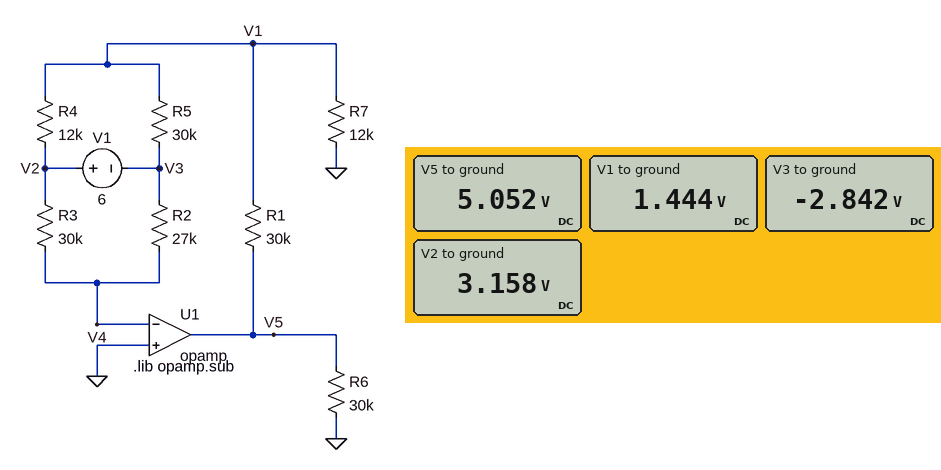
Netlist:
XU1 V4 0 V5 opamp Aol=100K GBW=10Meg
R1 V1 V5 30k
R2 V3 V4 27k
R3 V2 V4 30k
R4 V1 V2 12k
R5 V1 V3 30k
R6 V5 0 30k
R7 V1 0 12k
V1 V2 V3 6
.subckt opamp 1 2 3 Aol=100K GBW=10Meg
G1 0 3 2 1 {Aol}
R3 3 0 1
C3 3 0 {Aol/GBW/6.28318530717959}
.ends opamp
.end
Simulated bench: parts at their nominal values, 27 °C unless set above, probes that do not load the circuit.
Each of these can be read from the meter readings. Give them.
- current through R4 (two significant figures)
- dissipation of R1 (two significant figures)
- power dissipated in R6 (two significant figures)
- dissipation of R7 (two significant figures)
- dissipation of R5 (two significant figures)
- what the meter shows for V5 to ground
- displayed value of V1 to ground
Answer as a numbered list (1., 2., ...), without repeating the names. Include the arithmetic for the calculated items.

1. (3.158 V - 1.444 V) / 12 kΩ = 140 µA
2. (5.052 V - 1.444 V)^2 / 30 kΩ = 430 µW
3. (5.052 V)^2 / 30 kΩ = 850 µW
4. (1.444 V)^2 / 12 kΩ = 170 µW
5. (1.444 V - (-2.842 V))^2 / 30 kΩ = 610 µW
6. 5.052 V
7. 1.444 V
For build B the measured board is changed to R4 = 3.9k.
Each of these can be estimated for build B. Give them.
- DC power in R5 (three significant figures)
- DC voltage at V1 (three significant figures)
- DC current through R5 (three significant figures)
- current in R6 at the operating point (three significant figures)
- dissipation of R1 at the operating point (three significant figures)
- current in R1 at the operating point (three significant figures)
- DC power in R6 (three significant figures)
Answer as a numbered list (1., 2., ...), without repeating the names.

1. 940 µW
2. 2.47 V
3. 177 µA
4. 288 µA
5. 1.27 mW
6. 206 µA
7. 2.49 mW
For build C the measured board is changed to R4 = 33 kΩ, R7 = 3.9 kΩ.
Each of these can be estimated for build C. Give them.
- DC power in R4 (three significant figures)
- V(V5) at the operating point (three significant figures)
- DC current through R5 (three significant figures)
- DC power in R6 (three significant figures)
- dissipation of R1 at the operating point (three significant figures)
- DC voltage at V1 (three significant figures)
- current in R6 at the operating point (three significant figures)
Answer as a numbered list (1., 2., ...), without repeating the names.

1. 299 µW
2. 131 mV
3. 95.2 µA
4. 569 nW
5. 446 nW
6. 15.0 mV
7. 4.36 µA
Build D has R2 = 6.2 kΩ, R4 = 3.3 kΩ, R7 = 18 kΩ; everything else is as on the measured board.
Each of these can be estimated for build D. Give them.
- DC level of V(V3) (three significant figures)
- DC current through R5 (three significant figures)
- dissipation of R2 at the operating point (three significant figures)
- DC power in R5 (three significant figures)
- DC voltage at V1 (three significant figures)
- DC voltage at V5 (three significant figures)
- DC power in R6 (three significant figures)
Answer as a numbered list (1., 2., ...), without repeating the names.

1. -1.03 V
2. 180 µA
3. 170 µW
4. 974 µW
5. 4.38 V
6. 11.7 V
7. 4.54 mW
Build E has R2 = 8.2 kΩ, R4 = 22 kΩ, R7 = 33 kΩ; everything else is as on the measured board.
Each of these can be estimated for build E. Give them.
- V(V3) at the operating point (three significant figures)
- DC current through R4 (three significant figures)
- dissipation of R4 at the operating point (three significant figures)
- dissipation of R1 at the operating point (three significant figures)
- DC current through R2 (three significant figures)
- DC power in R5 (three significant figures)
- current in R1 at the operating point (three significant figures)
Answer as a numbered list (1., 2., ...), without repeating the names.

1. -1.29 V
2. 115 µA
3. 293 µW
4. 130 µW
5. 157 µA
6. 399 µW
7. 65.9 µA
